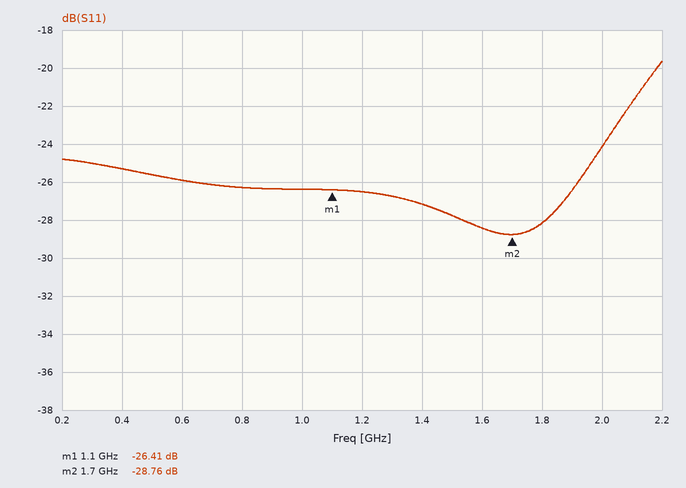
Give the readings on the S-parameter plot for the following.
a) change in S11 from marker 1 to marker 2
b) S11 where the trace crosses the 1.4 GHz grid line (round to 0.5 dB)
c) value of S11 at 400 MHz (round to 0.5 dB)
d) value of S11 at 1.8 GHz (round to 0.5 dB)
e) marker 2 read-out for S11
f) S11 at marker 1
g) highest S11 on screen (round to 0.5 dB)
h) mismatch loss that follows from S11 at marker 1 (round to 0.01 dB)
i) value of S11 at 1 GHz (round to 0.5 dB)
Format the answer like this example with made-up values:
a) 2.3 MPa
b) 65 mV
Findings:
a) -2.35 dB
b) -27.0 dB
c) -25.5 dB
d) -28.0 dB
e) -28.76 dB
f) -26.41 dB
g) -19.5 dB
h) 0.01 dB
i) -26.5 dB
